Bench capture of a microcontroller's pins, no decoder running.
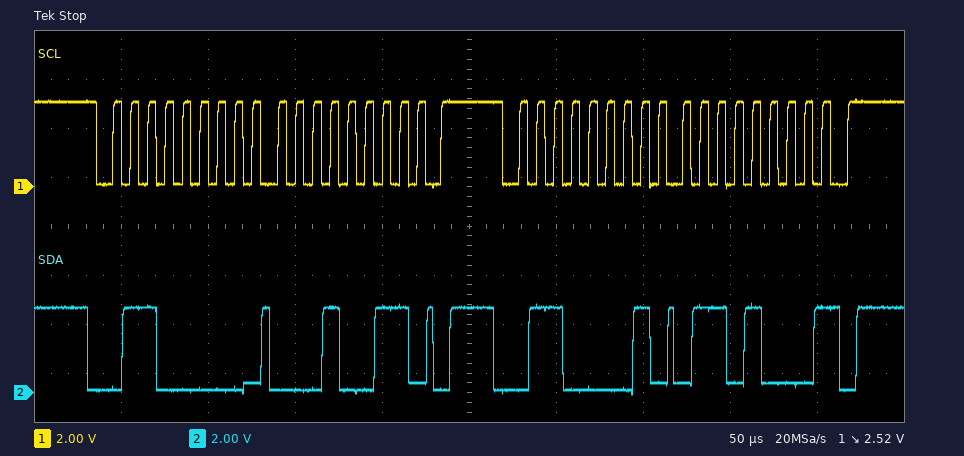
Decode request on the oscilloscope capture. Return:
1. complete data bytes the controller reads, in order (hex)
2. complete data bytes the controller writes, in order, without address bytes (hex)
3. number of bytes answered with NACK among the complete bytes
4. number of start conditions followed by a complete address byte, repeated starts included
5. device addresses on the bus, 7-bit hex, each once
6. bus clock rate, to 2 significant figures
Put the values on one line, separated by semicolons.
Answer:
68; 13; 1; 2; 0x30; 100 kHz
